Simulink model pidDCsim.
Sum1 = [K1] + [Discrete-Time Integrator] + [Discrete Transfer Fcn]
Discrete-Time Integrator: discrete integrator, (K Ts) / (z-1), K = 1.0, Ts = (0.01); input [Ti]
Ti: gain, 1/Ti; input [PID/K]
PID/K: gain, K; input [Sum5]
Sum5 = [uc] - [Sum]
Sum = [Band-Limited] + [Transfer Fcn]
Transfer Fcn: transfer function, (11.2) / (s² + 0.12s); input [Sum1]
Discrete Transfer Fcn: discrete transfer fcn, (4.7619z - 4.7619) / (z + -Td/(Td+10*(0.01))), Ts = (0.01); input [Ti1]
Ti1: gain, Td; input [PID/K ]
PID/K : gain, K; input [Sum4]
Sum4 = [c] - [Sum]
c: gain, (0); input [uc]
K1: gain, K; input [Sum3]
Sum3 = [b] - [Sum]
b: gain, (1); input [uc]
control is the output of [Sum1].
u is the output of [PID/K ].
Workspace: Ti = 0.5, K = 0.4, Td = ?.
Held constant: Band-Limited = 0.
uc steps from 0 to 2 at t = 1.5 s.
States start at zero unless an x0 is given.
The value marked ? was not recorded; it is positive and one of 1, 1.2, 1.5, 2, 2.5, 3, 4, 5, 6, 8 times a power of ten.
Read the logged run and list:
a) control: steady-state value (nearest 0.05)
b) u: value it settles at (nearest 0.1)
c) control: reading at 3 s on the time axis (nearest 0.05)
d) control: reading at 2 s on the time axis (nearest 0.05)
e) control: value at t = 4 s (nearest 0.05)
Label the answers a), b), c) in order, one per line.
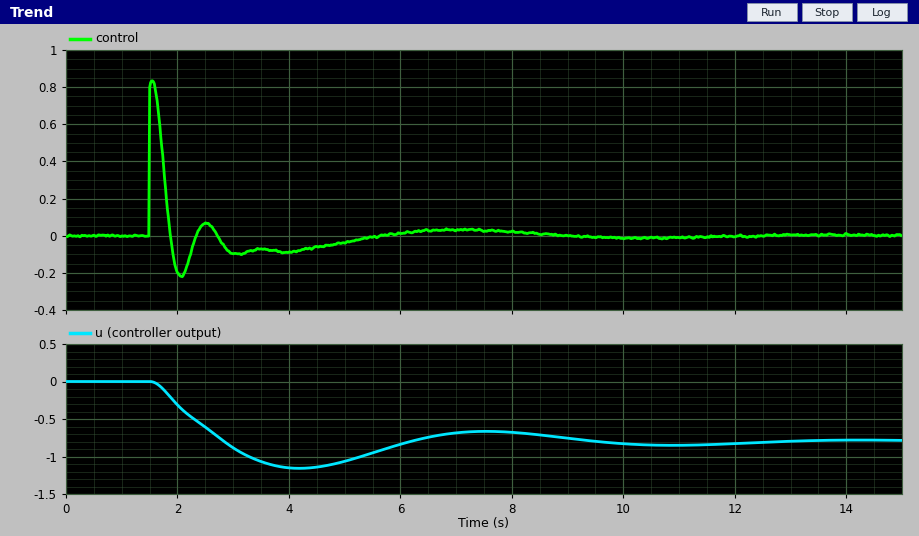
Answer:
a) 0.00
b) -0.8
c) -0.10
d) -0.20
e) -0.10
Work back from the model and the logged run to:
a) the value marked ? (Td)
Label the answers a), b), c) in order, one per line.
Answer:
a) 2
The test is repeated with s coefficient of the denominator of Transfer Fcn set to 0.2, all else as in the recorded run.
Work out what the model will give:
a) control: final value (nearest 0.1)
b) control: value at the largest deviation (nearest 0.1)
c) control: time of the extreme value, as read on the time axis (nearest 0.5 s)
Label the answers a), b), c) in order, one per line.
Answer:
a) 0.0
b) 0.8
c) 1.5 s
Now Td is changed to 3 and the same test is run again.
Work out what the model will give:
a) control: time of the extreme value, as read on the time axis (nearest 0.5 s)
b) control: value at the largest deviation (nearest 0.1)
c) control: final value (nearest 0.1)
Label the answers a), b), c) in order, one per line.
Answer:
a) 1.5 s
b) 0.8
c) 0.0
